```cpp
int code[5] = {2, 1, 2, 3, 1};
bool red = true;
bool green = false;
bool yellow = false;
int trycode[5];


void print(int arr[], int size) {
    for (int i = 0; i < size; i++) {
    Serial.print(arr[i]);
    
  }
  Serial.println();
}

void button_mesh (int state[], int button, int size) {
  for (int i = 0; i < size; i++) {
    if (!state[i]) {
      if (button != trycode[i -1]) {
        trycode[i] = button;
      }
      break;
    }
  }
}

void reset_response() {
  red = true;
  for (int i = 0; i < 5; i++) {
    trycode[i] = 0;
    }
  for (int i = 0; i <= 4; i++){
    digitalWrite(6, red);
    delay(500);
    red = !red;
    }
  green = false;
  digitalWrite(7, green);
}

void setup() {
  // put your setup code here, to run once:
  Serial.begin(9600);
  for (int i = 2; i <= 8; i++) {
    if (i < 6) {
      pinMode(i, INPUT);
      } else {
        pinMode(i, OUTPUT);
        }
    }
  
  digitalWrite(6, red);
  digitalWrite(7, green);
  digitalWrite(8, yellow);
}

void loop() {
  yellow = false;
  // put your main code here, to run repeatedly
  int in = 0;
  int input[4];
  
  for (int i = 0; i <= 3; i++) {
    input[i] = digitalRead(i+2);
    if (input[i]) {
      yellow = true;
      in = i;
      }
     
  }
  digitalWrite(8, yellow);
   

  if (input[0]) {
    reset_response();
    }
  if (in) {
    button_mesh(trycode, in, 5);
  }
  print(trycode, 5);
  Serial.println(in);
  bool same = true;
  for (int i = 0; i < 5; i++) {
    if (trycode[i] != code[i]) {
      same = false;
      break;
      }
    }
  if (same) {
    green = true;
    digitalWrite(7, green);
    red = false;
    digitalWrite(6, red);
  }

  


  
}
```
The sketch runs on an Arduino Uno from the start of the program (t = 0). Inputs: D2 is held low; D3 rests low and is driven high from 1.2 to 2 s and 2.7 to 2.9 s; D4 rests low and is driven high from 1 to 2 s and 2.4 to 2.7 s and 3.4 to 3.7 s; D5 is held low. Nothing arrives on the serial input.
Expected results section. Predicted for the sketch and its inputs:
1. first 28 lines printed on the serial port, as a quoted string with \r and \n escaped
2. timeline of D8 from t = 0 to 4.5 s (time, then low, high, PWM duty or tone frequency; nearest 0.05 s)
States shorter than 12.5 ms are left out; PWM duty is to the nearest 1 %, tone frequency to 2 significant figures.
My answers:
"00000\r\n0\r\n00000\r\n0\r\n00000\r\n0\r\n00000\r\n0\r\n00000\r\n0\r\n00000\r\n0\r\n00000\r\n0\r\n00000\r\n0\r\n00000\r\n0\r\n00000\r\n0\r\n00000\r\n0\r\n00000\r\n0\r\n00000\r\n0\r\n00000\r\n0\r\n"
0 s low; 1 s high; 2 s low; 2.4 s high; 2.9 s low; 3.4 s high; 3.7 s low
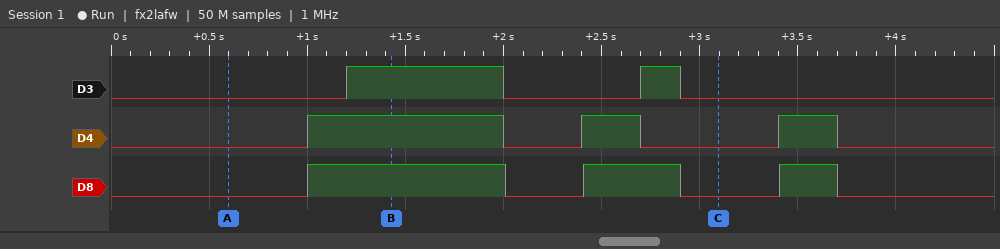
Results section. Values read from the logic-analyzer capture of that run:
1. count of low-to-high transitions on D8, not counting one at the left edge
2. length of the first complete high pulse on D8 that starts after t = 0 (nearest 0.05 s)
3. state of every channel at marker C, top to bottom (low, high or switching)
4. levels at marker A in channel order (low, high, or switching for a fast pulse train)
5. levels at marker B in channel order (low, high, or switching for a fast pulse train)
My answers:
3
1.00 s
D3 low, D4 low, D8 low
D3 low, D4 low, D8 low
D3 high, D4 high, D8 high
